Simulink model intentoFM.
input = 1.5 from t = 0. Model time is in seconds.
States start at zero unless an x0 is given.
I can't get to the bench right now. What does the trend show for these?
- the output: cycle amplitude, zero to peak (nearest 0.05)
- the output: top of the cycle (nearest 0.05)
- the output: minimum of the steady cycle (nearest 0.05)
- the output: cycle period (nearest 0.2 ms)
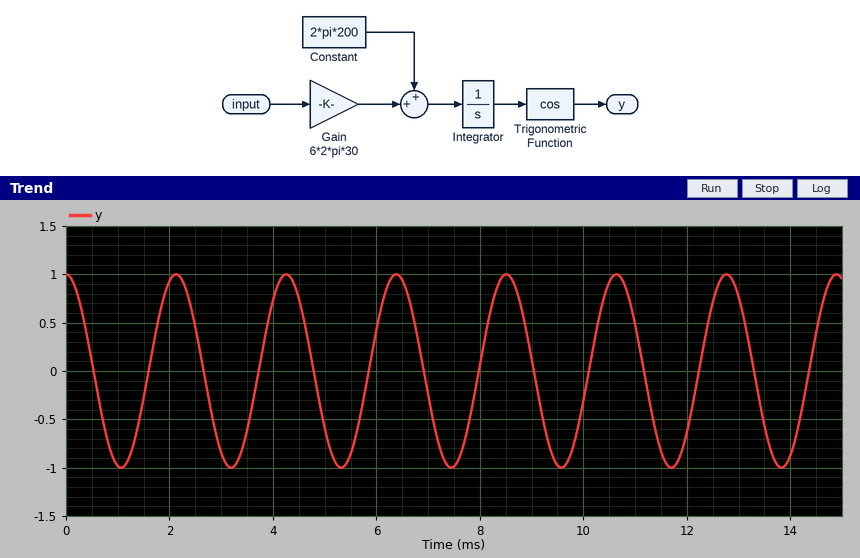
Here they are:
1.00
1.00
-1.00
2.2 ms
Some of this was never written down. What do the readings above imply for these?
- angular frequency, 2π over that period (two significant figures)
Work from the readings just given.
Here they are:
2.9 rad/ms
